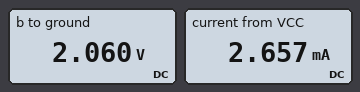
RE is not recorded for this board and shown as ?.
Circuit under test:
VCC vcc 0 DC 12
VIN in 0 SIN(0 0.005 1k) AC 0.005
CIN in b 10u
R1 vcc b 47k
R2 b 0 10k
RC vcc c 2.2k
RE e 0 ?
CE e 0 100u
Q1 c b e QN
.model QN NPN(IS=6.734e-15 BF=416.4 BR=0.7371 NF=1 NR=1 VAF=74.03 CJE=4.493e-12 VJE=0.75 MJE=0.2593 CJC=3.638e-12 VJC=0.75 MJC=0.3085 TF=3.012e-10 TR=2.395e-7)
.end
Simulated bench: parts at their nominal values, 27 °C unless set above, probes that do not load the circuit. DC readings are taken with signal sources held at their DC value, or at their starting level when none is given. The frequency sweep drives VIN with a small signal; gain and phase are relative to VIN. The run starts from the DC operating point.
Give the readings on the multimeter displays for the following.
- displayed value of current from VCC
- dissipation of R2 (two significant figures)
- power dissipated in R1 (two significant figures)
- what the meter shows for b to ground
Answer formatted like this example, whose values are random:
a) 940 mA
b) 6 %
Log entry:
a) 2.657 mA
b) 420 µW
c) 2.1 mW
d) 2.060 V
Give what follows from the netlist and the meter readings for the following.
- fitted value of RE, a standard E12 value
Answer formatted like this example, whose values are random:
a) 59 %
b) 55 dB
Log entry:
a) 560 Ω
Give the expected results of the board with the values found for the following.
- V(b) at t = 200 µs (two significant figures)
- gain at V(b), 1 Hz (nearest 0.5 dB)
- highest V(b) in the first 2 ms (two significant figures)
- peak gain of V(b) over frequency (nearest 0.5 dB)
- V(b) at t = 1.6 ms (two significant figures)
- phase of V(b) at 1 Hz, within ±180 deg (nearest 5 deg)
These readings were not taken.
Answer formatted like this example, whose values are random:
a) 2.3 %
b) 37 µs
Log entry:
a) 2.1 V
b) -7.0 dB
c) 2.1 V
d) 0 dB
e) 2.1 V
f) 65 deg
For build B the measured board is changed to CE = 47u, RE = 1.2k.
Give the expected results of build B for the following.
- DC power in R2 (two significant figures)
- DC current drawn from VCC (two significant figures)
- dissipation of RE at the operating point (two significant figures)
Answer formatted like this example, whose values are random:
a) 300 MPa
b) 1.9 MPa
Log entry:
a) 430 µW
b) 1.4 mA
c) 1.7 mW
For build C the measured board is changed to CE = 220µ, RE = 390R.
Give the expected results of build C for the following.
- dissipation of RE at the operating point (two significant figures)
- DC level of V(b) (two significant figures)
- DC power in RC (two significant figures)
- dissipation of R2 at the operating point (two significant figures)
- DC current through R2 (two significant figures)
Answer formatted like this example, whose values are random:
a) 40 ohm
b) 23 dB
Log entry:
a) 4.6 mW
b) 2.0 V
c) 26 mW
d) 420 µW
e) 200 µA
